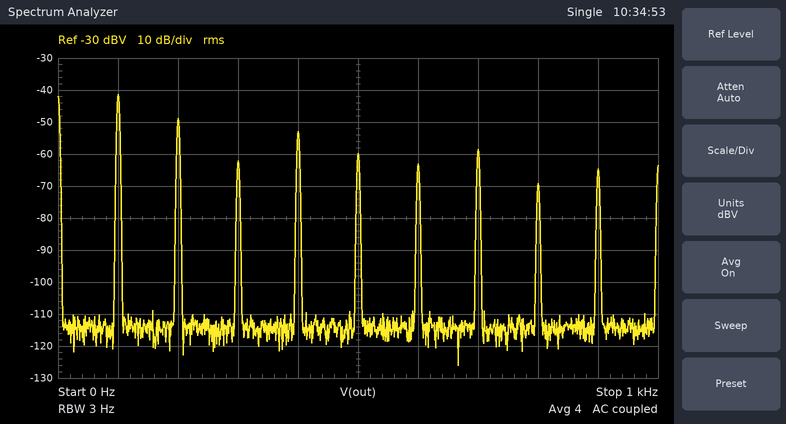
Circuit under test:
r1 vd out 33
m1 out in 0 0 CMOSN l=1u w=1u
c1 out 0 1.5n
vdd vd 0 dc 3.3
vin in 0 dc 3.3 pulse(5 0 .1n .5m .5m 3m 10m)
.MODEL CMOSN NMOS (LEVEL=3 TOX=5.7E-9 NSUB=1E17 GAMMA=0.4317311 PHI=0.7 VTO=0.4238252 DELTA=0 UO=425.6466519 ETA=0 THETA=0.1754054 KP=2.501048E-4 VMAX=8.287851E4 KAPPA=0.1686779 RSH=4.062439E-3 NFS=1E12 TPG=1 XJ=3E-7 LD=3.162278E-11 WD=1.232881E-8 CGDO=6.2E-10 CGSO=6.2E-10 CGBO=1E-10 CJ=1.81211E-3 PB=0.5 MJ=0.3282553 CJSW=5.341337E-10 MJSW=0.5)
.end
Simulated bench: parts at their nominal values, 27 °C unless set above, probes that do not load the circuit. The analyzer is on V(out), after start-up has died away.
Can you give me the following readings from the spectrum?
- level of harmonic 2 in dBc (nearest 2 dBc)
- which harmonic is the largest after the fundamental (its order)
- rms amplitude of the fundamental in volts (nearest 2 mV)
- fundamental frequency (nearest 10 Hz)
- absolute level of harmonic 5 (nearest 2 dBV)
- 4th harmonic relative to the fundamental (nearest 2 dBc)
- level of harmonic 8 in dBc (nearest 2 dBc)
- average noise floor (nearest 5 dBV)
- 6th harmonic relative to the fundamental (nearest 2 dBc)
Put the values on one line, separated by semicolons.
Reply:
-8 dBc; 2; 8 mV; 100 Hz; -60 dBV; -12 dBc; -28 dBc; -115 dBV; -22 dBc
